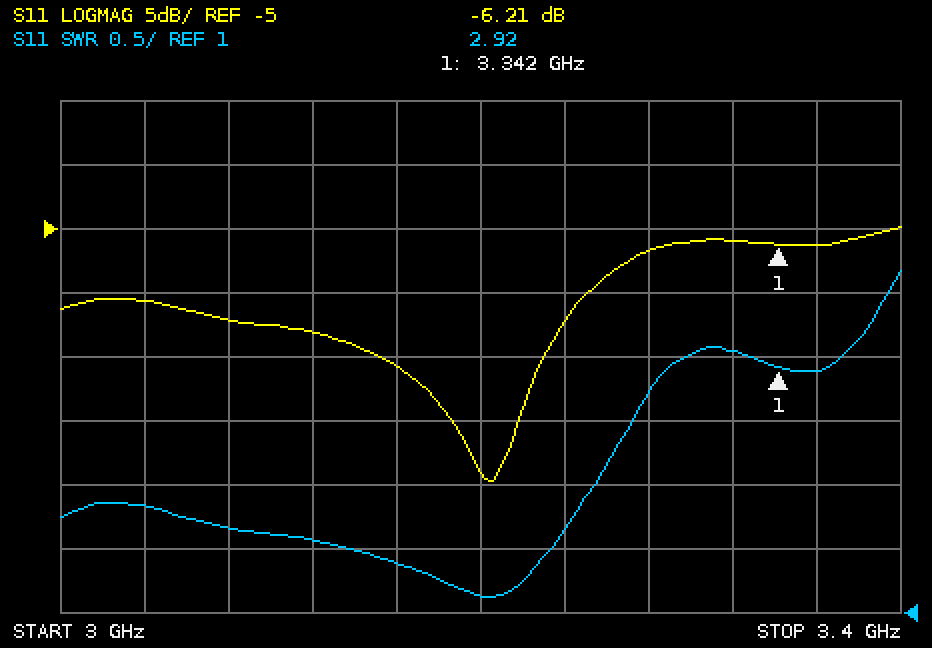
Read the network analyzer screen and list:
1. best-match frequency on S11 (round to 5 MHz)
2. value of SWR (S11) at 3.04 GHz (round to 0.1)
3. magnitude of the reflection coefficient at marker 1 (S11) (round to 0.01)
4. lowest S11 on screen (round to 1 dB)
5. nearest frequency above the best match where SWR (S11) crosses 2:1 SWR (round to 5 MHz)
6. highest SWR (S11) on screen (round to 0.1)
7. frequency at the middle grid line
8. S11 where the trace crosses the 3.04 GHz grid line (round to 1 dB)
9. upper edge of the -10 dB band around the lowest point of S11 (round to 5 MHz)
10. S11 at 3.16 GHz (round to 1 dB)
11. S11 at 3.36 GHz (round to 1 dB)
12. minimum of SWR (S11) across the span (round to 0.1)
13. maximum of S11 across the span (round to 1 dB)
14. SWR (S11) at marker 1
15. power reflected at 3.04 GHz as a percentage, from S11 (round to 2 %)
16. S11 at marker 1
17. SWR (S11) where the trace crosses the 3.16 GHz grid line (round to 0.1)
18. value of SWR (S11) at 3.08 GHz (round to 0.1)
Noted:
3.205 GHz
1.8
0.49
-25 dB
3.255 GHz
3.7
3.2 GHz
-11 dB
3.250 GHz
-16 dB
-6 dB
1.1
-5 dB
2.92
8 %
-6.21 dB
1.4
1.7
